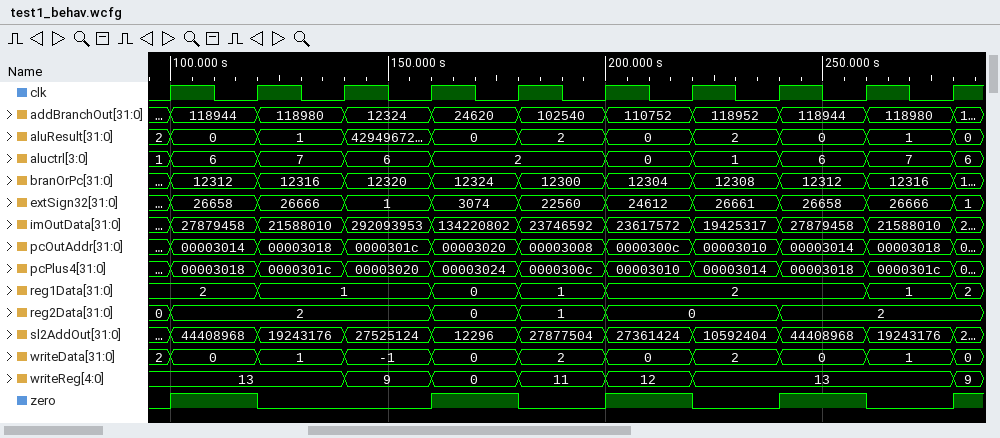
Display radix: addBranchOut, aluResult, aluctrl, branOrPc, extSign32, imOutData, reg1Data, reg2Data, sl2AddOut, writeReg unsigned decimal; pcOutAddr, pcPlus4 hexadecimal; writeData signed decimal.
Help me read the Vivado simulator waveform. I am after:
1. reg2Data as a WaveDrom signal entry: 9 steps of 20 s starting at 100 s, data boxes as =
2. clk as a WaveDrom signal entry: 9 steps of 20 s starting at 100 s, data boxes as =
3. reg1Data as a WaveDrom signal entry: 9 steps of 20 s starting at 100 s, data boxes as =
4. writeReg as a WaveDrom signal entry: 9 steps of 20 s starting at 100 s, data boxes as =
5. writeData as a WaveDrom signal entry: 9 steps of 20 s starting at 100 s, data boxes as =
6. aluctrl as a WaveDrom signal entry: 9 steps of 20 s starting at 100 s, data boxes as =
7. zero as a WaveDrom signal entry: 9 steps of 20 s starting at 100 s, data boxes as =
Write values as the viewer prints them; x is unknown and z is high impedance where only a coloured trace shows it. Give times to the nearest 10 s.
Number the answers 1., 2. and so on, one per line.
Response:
1. {name: 'reg2Data', wave: '=..===.=.', data: '2 0 1 0 2'}
2. {name: 'clk', wave: 'p........'}
3. {name: 'reg1Data', wave: '==.===..=', data: '2 1 0 1 2 1'}
4. {name: 'writeReg', wave: '=.=====..', data: '13 9 0 11 12 13'}
5. {name: 'writeData', wave: '=========', data: '0 1 -1 0 2 0 2 0 1'}
6. {name: 'aluctrl', wave: '====.====', data: '6 7 6 2 0 1 6 7'}
7. {name: 'zero', wave: '10.101010'}
